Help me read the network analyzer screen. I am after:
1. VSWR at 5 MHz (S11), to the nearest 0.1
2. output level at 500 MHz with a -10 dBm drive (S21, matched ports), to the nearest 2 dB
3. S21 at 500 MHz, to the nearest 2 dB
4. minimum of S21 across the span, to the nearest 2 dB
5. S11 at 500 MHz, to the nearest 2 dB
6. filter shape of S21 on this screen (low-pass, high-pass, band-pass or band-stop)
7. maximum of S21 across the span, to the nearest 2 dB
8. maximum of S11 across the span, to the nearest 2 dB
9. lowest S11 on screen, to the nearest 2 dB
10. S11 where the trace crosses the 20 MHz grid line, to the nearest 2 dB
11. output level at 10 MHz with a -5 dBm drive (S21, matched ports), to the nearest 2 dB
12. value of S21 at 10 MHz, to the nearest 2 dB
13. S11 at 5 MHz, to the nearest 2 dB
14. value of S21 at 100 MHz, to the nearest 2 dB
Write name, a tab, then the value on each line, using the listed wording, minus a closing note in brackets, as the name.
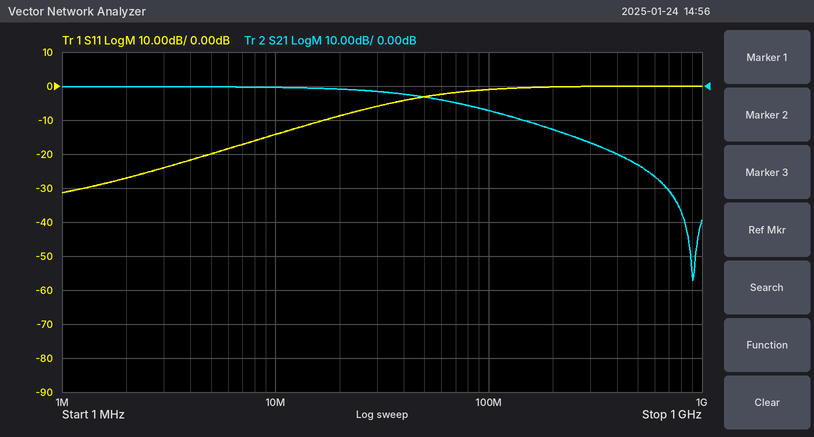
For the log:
VSWR at 5 MHz (S11), to the nearest 0.1	1.2
output level at 500 MHz with a -10 dBm drive (S21, matched ports), to the nearest 2 dB	-34 dBm
S21 at 500 MHz, to the nearest 2 dB	-24 dB
minimum of S21 across the span, to the nearest 2 dB	-58 dB
S11 at 500 MHz, to the nearest 2 dB	0 dB
filter shape of S21 on this screen	low-pass
maximum of S21 across the span, to the nearest 2 dB	0 dB
maximum of S11 across the span, to the nearest 2 dB	0 dB
lowest S11 on screen, to the nearest 2 dB	-32 dB
S11 where the trace crosses the 20 MHz grid line, to the nearest 2 dB	-8 dB
output level at 10 MHz with a -5 dBm drive (S21, matched ports), to the nearest 2 dB	-6 dBm
value of S21 at 10 MHz, to the nearest 2 dB	0 dB
S11 at 5 MHz, to the nearest 2 dB	-20 dB
value of S21 at 100 MHz, to the nearest 2 dB	-8 dB
